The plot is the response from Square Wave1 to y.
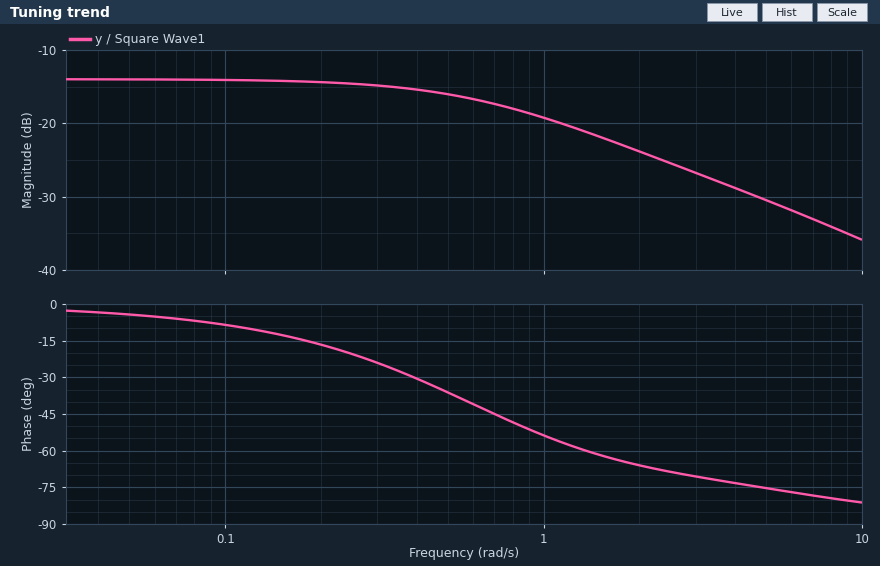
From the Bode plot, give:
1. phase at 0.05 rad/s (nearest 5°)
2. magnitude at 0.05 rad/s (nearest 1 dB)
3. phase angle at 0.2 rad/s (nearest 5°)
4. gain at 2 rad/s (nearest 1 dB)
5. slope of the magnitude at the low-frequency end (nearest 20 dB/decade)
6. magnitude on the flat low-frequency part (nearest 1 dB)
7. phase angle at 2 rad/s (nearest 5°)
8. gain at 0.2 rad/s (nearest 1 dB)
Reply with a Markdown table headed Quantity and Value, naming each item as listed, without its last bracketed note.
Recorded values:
| Quantity | Value |
|---|---|
| phase at 0.05 rad/s | -5° |
| magnitude at 0.05 rad/s | -14 dB |
| phase angle at 0.2 rad/s | -15° |
| gain at 2 rad/s | -24 dB |
| slope of the magnitude at the low-frequency end | 0 dB/decade |
| magnitude on the flat low-frequency part | -14 dB |
| phase angle at 2 rad/s | -65° |
| gain at 0.2 rad/s | -14 dB |
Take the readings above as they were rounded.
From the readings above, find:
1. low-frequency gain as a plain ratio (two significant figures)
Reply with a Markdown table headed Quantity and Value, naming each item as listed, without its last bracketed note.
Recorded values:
| Quantity | Value |
|---|---|
| low-frequency gain as a plain ratio | 0.20 |
